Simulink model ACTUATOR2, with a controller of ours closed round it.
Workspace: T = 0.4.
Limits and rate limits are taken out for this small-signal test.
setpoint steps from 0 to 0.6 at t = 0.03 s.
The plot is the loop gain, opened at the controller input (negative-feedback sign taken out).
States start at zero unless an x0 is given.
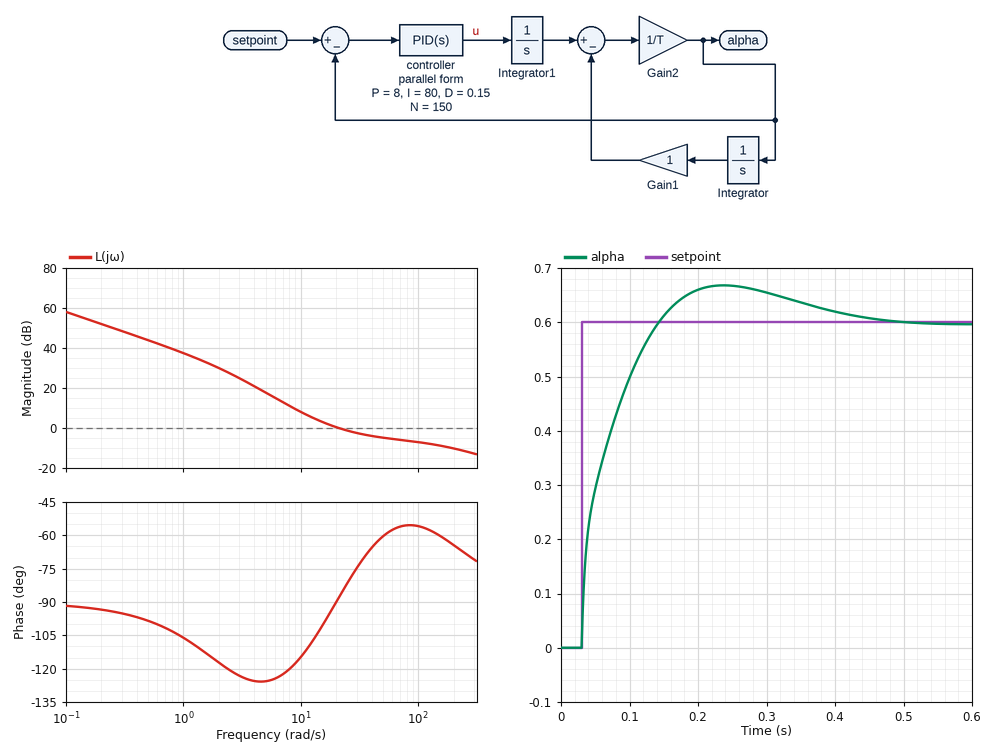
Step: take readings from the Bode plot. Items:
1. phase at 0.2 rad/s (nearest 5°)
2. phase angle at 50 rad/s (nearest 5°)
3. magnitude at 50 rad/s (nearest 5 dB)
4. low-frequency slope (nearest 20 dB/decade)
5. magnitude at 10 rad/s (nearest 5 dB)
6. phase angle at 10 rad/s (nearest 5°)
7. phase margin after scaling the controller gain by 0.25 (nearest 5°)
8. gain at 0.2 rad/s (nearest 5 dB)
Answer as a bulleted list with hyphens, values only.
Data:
- -95°
- -60°
- -5 dB
- -20 dB/decade
- 10 dB
- -115°
- 60°
- 50 dB
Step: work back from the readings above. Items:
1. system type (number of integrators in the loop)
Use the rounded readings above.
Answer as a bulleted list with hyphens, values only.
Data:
- 1
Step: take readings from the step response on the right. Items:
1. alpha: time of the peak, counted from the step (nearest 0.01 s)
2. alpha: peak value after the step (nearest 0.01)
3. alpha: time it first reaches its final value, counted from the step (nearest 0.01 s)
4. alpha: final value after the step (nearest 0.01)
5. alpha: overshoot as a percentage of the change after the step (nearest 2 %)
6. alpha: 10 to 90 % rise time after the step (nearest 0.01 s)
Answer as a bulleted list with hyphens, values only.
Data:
- 0.21 s
- 0.67
- 0.11 s
- 0.60
- 12 %
- 0.08 s
